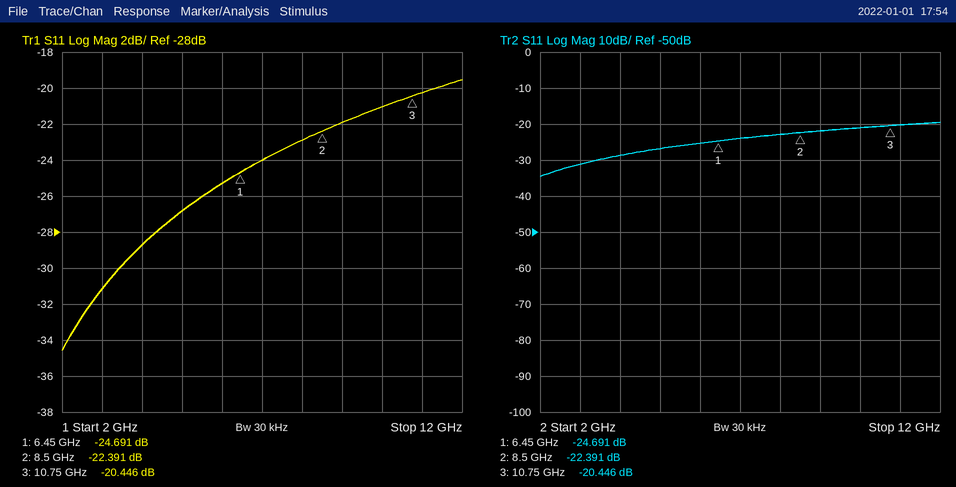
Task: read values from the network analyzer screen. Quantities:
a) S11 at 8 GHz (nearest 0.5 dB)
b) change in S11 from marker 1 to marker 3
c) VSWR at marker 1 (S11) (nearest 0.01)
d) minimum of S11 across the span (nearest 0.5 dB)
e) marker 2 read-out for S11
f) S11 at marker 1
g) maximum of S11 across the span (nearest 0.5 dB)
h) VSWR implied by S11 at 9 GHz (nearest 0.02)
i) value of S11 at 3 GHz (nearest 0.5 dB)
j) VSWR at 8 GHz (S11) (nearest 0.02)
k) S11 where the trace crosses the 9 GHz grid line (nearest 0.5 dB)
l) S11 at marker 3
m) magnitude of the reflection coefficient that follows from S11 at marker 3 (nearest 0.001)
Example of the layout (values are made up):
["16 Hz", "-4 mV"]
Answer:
["-23.0 dB", "4.245 dB", "1.12", "-34.5 dB", "-22.391 dB", "-24.691 dB", "-19.5 dB", "1.18", "-31.0 dB", "1.16", "-22.0 dB", "-20.446 dB", "0.095"]
